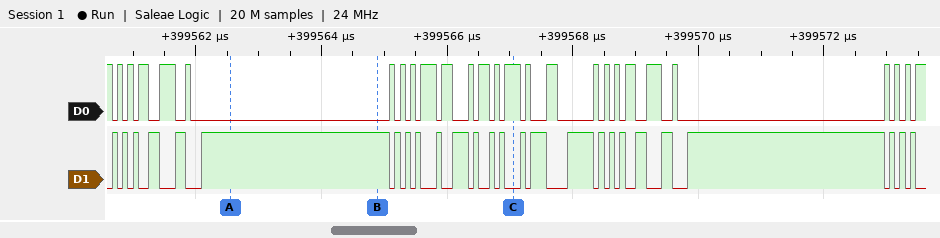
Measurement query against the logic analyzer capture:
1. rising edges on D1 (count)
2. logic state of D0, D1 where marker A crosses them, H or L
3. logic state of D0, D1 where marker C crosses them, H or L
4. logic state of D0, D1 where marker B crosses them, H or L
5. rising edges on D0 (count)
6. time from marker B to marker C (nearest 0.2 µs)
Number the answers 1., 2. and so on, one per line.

1. 26
2. D0=L, D1=H
3. D0=H, D1=L
4. D0=L, D1=H
5. 26
6. 2.2 µs
